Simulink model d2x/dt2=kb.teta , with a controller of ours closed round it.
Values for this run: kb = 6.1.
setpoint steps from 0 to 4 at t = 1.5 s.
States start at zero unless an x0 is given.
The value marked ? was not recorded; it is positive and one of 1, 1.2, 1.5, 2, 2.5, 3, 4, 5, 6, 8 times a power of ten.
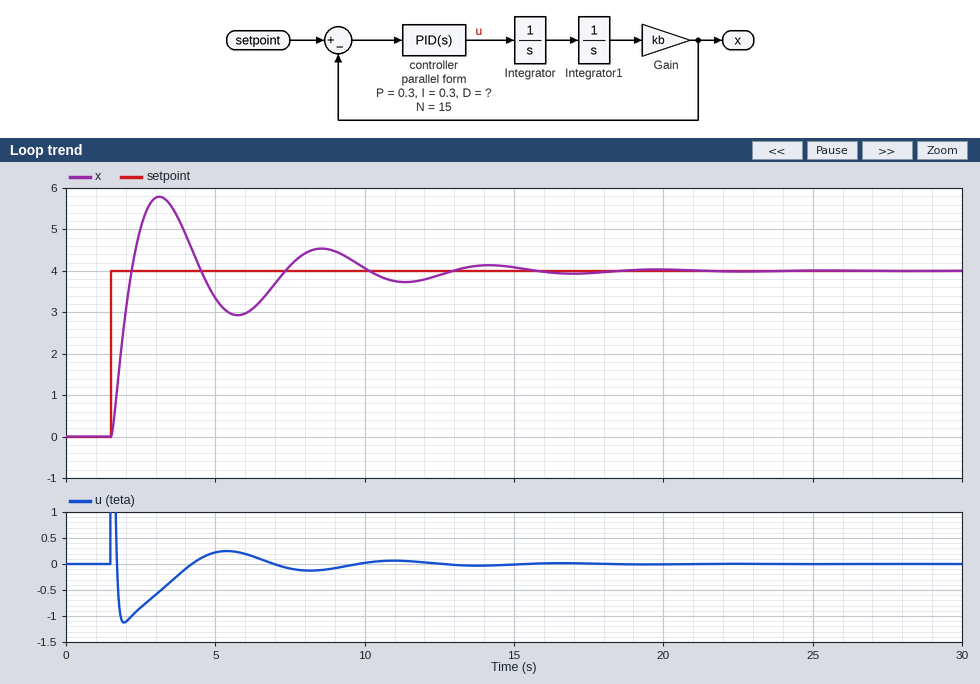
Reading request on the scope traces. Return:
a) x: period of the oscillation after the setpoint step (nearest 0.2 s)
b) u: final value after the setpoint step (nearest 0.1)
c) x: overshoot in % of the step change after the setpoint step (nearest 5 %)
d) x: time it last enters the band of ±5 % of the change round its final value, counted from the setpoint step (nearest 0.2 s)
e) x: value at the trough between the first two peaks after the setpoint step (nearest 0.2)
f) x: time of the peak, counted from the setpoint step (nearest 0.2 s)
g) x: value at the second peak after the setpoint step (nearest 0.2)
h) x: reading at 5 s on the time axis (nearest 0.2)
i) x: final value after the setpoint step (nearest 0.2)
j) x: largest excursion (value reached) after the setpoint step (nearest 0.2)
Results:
5.4 s
0.0
45 %
10.6 s
3.0
1.6 s
4.6
3.4
4.0
5.8
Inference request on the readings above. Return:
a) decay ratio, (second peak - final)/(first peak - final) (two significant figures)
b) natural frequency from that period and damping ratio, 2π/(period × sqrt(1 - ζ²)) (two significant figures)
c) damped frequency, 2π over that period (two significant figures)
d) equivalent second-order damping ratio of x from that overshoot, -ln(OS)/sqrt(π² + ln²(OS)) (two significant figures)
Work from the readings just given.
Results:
0.33
1.2 rad/s
1.2 rad/s
0.25
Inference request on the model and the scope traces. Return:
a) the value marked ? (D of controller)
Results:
0.3
